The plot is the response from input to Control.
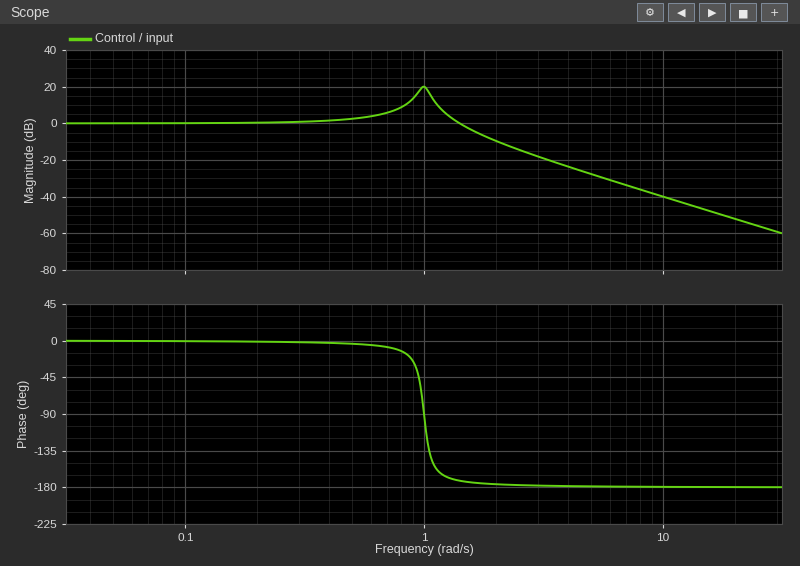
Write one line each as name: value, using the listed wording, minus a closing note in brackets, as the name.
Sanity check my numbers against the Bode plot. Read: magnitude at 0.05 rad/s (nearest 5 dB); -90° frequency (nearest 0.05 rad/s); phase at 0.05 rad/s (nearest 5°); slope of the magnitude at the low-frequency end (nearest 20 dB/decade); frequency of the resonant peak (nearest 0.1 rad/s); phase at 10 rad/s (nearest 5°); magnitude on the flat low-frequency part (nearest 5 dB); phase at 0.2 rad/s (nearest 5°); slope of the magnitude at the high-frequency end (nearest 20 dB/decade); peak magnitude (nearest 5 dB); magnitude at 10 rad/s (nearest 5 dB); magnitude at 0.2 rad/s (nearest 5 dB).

magnitude at 0.05 rad/s: 0 dB
-90° frequency: 1.00 rad/s
phase at 0.05 rad/s: 0°
slope of the magnitude at the low-frequency end: 0 dB/decade
frequency of the resonant peak: 1.0 rad/s
phase at 10 rad/s: -180°
magnitude on the flat low-frequency part: 0 dB
phase at 0.2 rad/s: 0°
slope of the magnitude at the high-frequency end: -40 dB/decade
peak magnitude: 20 dB
magnitude at 10 rad/s: -40 dB
magnitude at 0.2 rad/s: 0 dB
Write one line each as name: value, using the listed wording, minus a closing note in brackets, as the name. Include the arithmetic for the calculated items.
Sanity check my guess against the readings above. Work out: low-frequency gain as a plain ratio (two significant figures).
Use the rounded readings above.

low-frequency gain as a plain ratio: 10^(0 / 20) = 1.0
